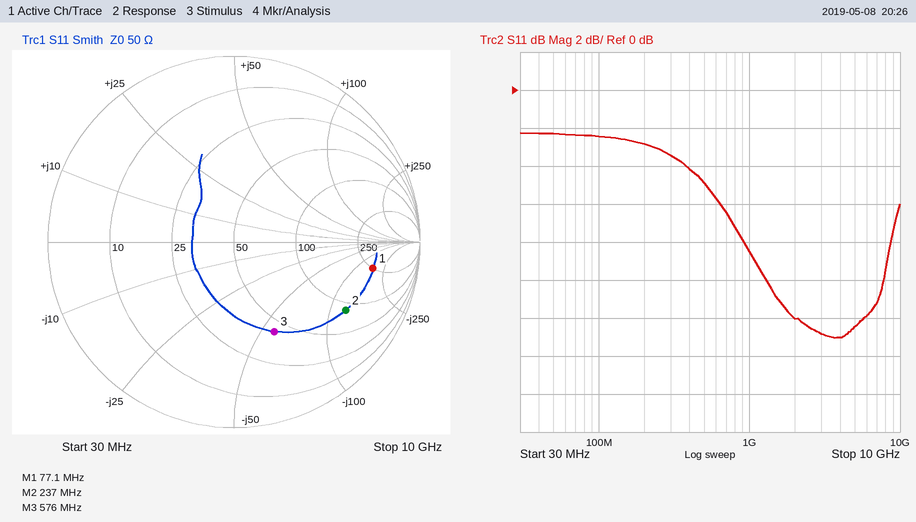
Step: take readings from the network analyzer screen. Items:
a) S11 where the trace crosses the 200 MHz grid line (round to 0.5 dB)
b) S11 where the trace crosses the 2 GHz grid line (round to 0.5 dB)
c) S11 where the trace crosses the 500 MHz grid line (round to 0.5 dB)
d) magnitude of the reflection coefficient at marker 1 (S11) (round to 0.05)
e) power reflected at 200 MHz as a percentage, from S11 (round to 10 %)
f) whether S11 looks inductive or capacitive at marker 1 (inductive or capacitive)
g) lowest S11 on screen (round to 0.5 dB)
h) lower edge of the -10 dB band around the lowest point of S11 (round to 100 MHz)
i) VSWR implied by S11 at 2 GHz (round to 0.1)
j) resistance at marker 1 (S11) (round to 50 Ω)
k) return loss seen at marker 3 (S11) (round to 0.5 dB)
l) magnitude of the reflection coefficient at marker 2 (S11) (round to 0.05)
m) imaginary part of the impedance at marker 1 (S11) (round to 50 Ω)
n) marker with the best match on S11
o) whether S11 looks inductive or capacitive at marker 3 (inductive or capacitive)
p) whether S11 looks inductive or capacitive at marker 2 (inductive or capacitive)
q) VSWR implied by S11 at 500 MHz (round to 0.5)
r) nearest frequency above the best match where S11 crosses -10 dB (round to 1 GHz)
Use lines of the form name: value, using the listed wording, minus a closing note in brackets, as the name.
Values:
S11 where the trace crosses the 200 MHz grid line: -3.0 dB
S11 where the trace crosses the 2 GHz grid line: -12.0 dB
S11 where the trace crosses the 500 MHz grid line: -5.0 dB
magnitude of the reflection coefficient at marker 1 (S11): 0.75
power reflected at 200 MHz as a percentage, from S11: 50 %
whether S11 looks inductive or capacitive at marker 1: capacitive
lowest S11 on screen: -13.0 dB
lower edge of the -10 dB band around the lowest point of S11: 1.3 GHz
VSWR implied by S11 at 2 GHz: 1.7
resistance at marker 1 (S11): 250 Ω
return loss seen at marker 3 (S11): 5.5 dB
magnitude of the reflection coefficient at marker 2 (S11): 0.70
imaginary part of the impedance at marker 1 (S11): -150 Ω
marker with the best match on S11: marker 3
whether S11 looks inductive or capacitive at marker 3: capacitive
whether S11 looks inductive or capacitive at marker 2: capacitive
VSWR implied by S11 at 500 MHz: 3.5
nearest frequency above the best match where S11 crosses -10 dB: 8 GHz
